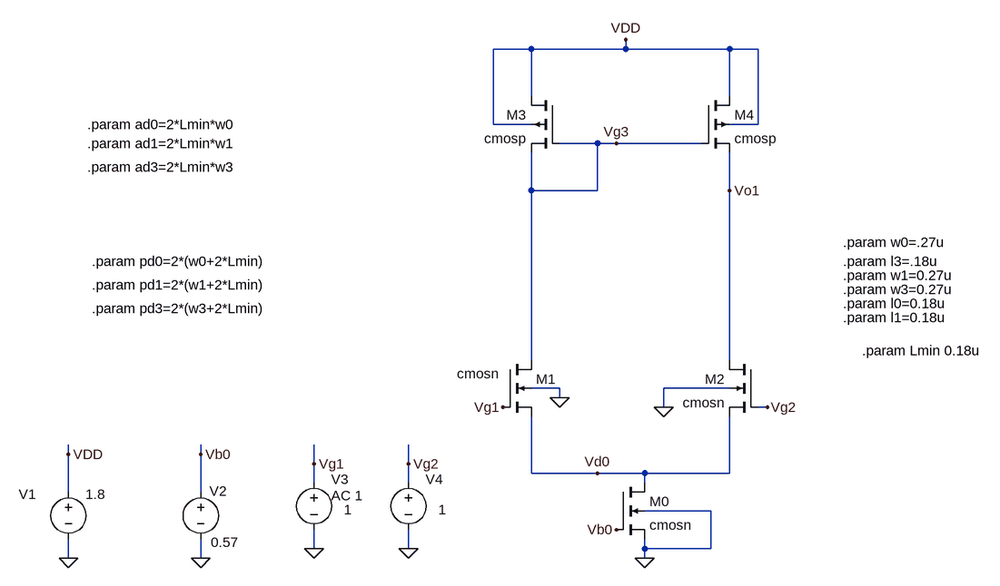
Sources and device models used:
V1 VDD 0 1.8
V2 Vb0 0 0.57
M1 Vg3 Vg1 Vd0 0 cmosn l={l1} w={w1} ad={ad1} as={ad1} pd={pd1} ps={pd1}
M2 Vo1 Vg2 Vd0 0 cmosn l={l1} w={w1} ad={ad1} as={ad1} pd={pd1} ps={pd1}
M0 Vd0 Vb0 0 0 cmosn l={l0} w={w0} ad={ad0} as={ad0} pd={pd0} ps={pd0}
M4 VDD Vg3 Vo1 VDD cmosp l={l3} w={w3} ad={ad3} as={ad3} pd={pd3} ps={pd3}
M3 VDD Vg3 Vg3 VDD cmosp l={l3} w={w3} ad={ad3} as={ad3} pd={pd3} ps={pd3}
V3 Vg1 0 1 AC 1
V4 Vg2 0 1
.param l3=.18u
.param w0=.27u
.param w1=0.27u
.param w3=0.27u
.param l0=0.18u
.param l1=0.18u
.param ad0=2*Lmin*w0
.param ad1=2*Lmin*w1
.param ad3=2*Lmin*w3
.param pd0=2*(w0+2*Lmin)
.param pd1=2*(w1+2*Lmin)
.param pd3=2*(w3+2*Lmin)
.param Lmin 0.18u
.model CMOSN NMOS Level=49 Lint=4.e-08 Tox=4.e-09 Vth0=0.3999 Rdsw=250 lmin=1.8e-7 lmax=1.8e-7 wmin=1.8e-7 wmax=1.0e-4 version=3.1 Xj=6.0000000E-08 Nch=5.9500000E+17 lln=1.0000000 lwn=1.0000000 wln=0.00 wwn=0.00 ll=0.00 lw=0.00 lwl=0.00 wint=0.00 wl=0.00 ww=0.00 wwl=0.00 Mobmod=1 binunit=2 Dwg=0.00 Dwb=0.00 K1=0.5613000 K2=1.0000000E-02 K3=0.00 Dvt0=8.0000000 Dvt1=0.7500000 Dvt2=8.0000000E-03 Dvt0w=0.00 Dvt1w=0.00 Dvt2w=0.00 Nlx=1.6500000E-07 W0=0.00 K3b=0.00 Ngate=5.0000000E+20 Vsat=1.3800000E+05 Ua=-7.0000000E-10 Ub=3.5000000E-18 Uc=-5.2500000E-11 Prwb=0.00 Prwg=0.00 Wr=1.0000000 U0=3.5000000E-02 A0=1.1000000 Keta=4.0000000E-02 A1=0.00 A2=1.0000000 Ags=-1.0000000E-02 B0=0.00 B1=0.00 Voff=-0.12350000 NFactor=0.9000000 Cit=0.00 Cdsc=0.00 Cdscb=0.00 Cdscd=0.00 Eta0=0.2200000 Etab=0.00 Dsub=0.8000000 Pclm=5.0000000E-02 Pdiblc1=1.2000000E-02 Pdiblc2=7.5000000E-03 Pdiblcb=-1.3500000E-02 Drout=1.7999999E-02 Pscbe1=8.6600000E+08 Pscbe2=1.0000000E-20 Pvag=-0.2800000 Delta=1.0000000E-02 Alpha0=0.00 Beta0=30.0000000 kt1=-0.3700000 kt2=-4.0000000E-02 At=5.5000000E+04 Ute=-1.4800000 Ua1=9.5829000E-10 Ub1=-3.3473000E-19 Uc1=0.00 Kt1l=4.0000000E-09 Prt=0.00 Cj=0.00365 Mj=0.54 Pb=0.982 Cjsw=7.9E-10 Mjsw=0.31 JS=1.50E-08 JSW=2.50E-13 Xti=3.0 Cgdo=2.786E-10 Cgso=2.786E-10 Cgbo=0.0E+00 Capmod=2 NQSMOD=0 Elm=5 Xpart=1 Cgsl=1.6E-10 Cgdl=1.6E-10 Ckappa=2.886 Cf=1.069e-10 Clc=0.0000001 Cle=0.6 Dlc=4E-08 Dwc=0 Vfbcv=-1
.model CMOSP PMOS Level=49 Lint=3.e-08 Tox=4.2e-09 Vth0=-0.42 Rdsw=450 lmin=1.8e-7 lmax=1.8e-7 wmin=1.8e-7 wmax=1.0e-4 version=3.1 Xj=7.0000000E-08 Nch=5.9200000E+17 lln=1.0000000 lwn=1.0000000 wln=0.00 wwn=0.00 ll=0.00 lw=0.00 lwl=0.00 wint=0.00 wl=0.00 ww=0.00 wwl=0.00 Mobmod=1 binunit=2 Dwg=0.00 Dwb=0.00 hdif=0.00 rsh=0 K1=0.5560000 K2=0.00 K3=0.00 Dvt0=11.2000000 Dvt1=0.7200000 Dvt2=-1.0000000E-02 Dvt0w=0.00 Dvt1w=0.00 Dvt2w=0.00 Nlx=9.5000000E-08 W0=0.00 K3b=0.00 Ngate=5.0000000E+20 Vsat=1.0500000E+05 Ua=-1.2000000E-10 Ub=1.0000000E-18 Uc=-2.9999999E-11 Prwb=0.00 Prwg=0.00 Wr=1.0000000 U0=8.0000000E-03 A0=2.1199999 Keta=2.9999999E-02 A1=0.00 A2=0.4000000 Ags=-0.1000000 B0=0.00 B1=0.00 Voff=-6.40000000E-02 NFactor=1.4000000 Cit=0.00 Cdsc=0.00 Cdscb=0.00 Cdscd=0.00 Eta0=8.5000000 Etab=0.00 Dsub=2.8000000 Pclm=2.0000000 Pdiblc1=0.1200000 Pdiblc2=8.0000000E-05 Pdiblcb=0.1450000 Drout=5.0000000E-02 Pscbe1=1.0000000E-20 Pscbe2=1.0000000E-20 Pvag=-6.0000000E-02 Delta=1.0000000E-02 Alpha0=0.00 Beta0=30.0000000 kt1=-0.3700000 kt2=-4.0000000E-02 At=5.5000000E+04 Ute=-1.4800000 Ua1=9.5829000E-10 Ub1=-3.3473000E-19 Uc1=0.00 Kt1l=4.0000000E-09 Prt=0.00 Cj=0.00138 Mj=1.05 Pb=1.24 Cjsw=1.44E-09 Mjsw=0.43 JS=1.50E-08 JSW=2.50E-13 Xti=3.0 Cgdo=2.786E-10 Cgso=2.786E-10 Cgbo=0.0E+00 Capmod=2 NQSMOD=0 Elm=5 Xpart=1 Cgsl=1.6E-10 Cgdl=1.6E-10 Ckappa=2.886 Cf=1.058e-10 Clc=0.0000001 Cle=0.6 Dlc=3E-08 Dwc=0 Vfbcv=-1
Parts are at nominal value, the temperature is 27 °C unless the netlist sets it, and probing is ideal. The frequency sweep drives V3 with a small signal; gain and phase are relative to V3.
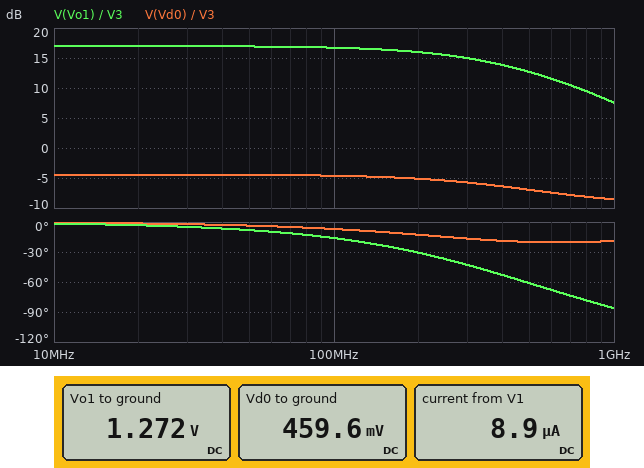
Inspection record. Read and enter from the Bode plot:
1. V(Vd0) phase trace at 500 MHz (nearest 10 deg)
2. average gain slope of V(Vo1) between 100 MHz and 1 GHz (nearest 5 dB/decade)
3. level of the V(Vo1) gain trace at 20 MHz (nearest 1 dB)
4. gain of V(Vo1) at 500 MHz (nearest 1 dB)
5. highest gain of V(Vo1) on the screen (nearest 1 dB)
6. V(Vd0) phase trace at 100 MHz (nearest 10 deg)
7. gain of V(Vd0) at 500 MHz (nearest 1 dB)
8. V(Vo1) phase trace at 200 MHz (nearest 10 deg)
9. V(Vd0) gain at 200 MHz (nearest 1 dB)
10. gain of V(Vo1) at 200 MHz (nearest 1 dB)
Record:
-20 deg
-10 dB/decade
17 dB
13 dB
17 dB
-10 deg
-7 dB
-30 deg
-5 dB
16 dB
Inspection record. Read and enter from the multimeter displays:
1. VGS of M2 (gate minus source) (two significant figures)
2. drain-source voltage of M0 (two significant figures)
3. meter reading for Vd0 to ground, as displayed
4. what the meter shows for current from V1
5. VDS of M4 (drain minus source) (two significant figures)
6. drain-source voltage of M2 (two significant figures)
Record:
540 mV
460 mV
459.6 mV
8.9 µA
530 mV
810 mV
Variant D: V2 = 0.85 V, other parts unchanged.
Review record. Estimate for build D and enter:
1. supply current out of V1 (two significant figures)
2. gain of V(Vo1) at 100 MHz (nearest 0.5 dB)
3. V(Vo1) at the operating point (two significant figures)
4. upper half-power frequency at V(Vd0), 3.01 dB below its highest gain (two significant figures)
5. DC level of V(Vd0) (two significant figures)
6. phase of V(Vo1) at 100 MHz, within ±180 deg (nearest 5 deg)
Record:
36 µA
14.5 dB
980 mV
1.4 GHz
310 mV
-5 deg
